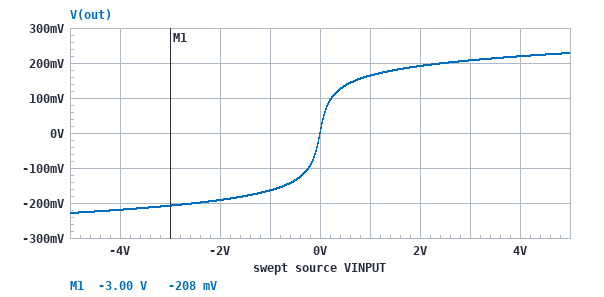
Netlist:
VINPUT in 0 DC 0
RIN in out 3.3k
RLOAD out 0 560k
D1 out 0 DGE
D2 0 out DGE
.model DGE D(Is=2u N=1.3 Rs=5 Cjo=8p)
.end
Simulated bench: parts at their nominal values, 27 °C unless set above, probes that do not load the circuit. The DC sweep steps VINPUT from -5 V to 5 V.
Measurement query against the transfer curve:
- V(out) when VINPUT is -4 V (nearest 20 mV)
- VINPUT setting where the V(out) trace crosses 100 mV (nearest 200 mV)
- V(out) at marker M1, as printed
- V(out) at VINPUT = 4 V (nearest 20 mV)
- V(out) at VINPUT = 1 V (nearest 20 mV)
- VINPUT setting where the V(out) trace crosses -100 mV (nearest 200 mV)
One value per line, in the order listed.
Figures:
-220 mV
200 mV
-208 mV
220 mV
160 mV
-200 mV
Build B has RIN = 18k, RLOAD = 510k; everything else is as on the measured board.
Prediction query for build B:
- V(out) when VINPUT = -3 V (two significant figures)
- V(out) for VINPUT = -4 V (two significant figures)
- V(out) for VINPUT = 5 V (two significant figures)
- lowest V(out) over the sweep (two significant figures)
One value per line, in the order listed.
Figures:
-150 mV
-160 mV
170 mV
-170 mV
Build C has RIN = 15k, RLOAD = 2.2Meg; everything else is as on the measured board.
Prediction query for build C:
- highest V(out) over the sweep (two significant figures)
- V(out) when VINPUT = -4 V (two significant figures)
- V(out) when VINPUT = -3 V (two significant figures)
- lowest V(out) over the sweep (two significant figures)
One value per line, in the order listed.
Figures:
170 mV
-160 mV
-150 mV
-170 mV
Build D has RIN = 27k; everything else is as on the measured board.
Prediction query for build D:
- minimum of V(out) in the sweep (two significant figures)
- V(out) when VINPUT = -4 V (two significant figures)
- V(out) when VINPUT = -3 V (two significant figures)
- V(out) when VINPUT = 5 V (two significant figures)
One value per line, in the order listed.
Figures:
-150 mV
-140 mV
-130 mV
150 mV
